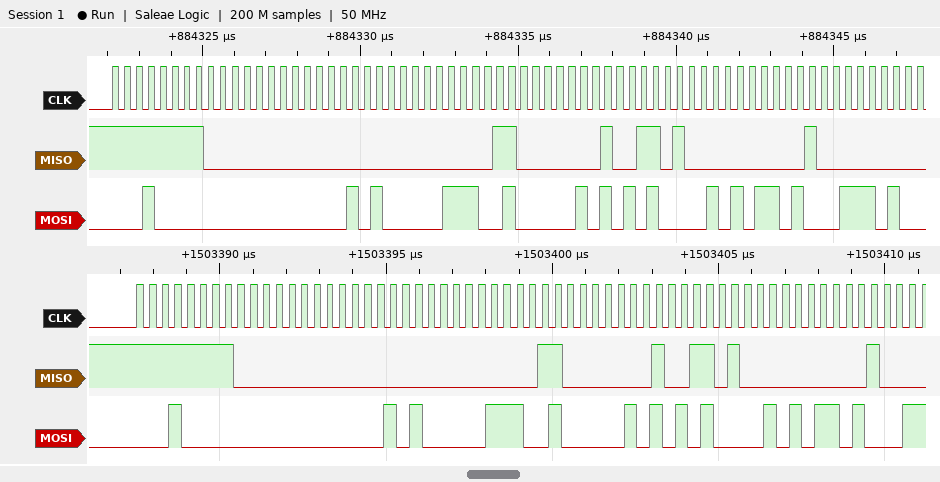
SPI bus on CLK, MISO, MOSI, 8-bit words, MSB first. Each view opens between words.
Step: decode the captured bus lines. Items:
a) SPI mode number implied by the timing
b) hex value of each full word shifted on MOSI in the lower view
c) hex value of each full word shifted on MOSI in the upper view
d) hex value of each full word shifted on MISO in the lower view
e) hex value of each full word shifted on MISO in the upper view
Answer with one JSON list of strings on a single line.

["0", "10, 00, 0A, 0E, 41, 54, 2B", "10, 00, 0A, 0E, 41, 54, 2B, 47", "FF, 00, 00, 00, C0, 4D, 00", "FF, 00, 00, 00, C0, 4D, 00, 20"]
